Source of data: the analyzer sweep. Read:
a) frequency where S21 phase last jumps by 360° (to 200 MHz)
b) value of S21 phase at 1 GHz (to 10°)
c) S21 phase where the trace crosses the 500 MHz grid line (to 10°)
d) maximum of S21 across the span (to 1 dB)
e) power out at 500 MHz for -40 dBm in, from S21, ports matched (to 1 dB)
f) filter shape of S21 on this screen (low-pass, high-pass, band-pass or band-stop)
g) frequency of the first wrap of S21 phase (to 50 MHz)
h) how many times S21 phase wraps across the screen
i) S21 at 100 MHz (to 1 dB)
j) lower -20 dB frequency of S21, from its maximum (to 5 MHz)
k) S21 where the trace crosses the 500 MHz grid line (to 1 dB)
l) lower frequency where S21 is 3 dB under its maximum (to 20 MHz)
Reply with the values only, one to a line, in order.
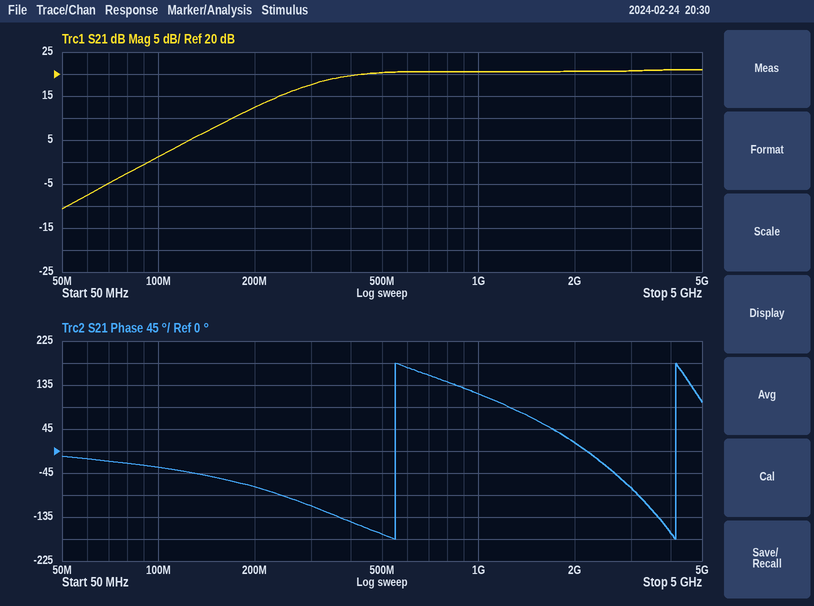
4.2 GHz
120°
-170°
21 dB
-20 dBm
high-pass
550 MHz
2
1 dB
100 MHz
20 dB
320 MHz
